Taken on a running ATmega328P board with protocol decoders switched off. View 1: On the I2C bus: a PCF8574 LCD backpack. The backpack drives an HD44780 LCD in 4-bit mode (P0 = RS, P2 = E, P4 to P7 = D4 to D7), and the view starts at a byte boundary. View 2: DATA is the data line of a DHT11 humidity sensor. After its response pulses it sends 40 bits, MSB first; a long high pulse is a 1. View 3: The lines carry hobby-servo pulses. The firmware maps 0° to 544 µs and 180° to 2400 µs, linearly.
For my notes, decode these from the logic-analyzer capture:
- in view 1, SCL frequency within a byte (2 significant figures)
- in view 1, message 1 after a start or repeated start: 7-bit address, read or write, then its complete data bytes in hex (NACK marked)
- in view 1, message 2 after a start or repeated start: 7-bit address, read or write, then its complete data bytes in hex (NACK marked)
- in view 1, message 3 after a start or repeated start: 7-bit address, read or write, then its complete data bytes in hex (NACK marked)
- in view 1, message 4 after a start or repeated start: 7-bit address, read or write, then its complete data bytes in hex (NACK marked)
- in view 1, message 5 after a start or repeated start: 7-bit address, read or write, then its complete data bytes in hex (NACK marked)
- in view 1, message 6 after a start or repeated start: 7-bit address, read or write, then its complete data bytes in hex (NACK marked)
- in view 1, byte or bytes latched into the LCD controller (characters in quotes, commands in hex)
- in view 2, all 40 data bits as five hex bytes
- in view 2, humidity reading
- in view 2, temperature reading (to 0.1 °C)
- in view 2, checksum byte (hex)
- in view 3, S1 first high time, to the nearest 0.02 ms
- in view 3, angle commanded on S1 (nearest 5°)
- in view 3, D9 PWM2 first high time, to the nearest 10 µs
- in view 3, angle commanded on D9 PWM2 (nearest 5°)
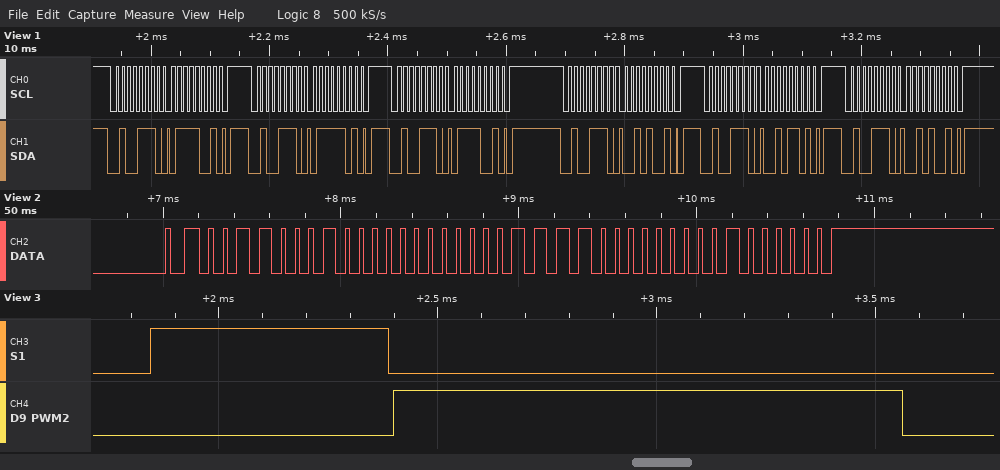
100 kHz
0x27 write: 79
0x27 write: 7D
0x27 write: 79
0x27 write: 29
0x27 write: 2D
0x27 write: 29
'r'
31 00 0F 00 40
49 %
15.0 °C
0x40
0.54 ms
0°
1160 µs
60°
